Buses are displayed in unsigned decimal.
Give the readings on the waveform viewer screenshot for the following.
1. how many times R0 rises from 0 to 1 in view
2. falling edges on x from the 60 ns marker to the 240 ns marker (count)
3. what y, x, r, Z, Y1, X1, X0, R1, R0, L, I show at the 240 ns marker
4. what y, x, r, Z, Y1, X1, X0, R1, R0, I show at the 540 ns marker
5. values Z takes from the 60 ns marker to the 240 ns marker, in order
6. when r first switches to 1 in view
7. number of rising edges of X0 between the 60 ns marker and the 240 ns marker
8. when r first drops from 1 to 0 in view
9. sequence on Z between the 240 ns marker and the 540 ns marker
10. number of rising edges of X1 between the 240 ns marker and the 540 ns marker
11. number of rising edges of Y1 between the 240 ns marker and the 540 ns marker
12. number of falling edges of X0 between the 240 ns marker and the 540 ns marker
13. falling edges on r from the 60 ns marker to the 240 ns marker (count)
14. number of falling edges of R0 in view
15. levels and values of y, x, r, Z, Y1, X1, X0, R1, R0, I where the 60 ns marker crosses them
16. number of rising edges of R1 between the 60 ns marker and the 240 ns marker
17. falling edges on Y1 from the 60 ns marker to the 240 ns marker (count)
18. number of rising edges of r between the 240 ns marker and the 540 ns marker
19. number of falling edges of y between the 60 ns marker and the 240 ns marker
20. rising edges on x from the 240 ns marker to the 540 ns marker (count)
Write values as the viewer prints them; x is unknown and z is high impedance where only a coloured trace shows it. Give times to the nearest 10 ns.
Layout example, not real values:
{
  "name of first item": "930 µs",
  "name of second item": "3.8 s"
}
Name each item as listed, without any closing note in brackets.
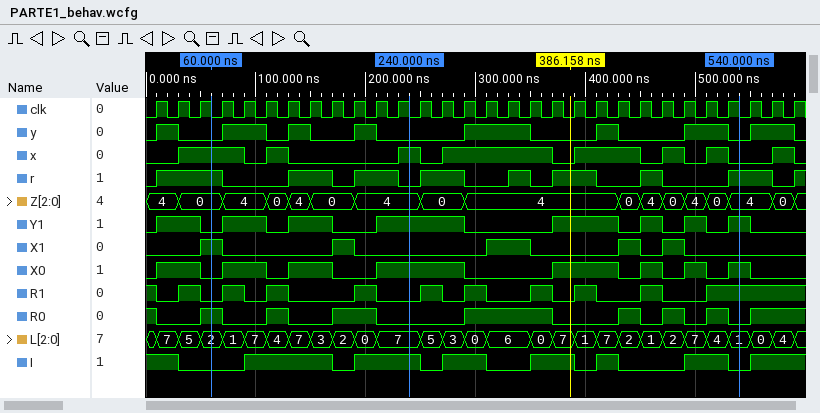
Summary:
{
  "how many times R0 rises from 0 to 1 in view": "8",
  "falling edges on x from the 60 ns marker to the 240 ns marker": "2",
  "what y, x, r, Z, Y1, X1, X0, R1, R0, L, I show at the 240 ns marker": "y=0, x=1, r=0, Z=4, Y1=1, X1=0, X0=1, R1=0, R0=0, L=7, I=1",
  "what y, x, r, Z, Y1, X1, X0, R1, R0, I show at the 540 ns marker": "y=0, x=0, r=1, Z=4, Y1=1, X1=0, X0=1, R1=1, R0=0, I=0",
  "values Z takes from the 60 ns marker to the 240 ns marker, in order": "0, 4, 0, 4, 0, 4",
  "when r first switches to 1 in view": "10 ns",
  "number of rising edges of X0 between the 60 ns marker and the 240 ns marker": "3",
  "when r first drops from 1 to 0 in view": "70 ns",
  "sequence on Z between the 240 ns marker and the 540 ns marker": "4, 0, 4, 0, 4, 0, 4, 0, 4",
  "number of rising edges of X1 between the 240 ns marker and the 540 ns marker": "3",
  "number of rising edges of Y1 between the 240 ns marker and the 540 ns marker": "4",
  "number of falling edges of X0 between the 240 ns marker and the 540 ns marker": "4",
  "falling edges on r from the 60 ns marker to the 240 ns marker": "3",
  "number of falling edges of R0 in view": "8",
  "levels and values of y, x, r, Z, Y1, X1, X0, R1, R0, I where the 60 ns marker crosses them": "y=0, x=1, r=1, Z=0, Y1=0, X1=1, X0=0, R1=0, R0=1, I=0",
  "number of rising edges of R1 between the 60 ns marker and the 240 ns marker": "3",
  "falling edges on Y1 from the 60 ns marker to the 240 ns marker": "2",
  "number of rising edges of r between the 240 ns marker and the 540 ns marker": "5",
  "number of falling edges of y between the 60 ns marker and the 240 ns marker": "3",
  "rising edges on x from the 240 ns marker to the 540 ns marker": "4"
}
